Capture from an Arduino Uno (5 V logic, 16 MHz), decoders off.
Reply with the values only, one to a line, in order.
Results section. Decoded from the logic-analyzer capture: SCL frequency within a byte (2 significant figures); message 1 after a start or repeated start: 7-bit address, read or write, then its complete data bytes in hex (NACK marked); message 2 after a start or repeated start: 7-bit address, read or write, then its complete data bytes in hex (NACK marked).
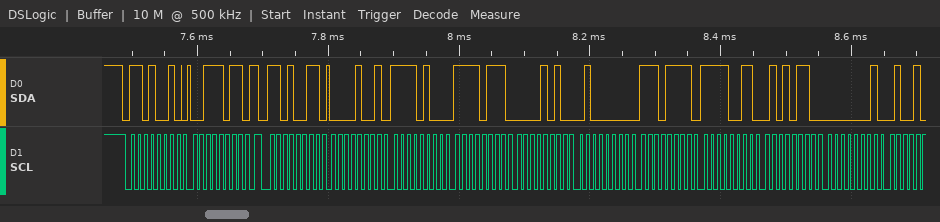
100 kHz
0x69 write: 3B
0x69 read: 09 F4 F7 0A 40 EF F3 56 01
